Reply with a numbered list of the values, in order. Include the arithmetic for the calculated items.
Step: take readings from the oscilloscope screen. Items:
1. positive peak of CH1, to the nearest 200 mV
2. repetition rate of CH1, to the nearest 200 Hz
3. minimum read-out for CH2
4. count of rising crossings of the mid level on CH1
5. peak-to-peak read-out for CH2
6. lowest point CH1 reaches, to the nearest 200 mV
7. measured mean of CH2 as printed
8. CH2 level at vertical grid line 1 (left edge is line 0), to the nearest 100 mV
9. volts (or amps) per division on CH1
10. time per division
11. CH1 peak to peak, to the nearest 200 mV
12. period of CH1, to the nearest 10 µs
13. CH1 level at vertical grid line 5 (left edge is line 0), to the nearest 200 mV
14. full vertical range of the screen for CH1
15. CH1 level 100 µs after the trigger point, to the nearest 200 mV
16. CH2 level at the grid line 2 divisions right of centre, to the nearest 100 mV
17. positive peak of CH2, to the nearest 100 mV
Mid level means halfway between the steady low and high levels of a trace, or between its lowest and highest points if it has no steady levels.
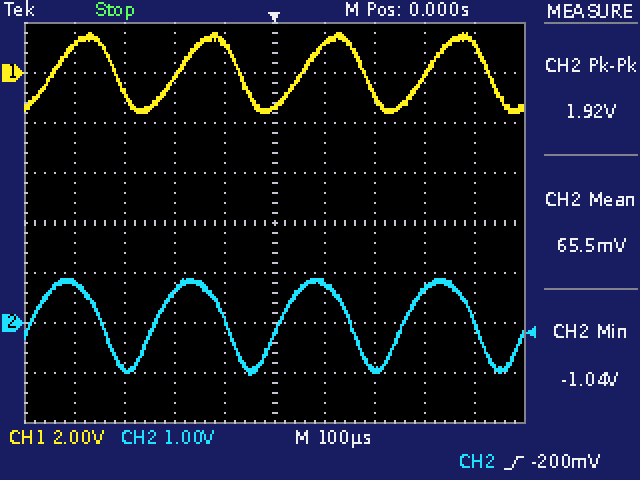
1. 1.6 V
2. 1 / 250 µs ≈ 4.0 kHz
3. -1.04 V
4. 4
5. 1.92 V
6. -1.6 V
7. 65.5 mV
8. 800 mV
9. 2 V
10. 100 µs
11. 1.6 V − (-1.6 V) = 3.2 V
12. 250 µs
13. -1.4 V
14. 16 V
15. 1.2 V
16. -900 mV
17. 900 mV
